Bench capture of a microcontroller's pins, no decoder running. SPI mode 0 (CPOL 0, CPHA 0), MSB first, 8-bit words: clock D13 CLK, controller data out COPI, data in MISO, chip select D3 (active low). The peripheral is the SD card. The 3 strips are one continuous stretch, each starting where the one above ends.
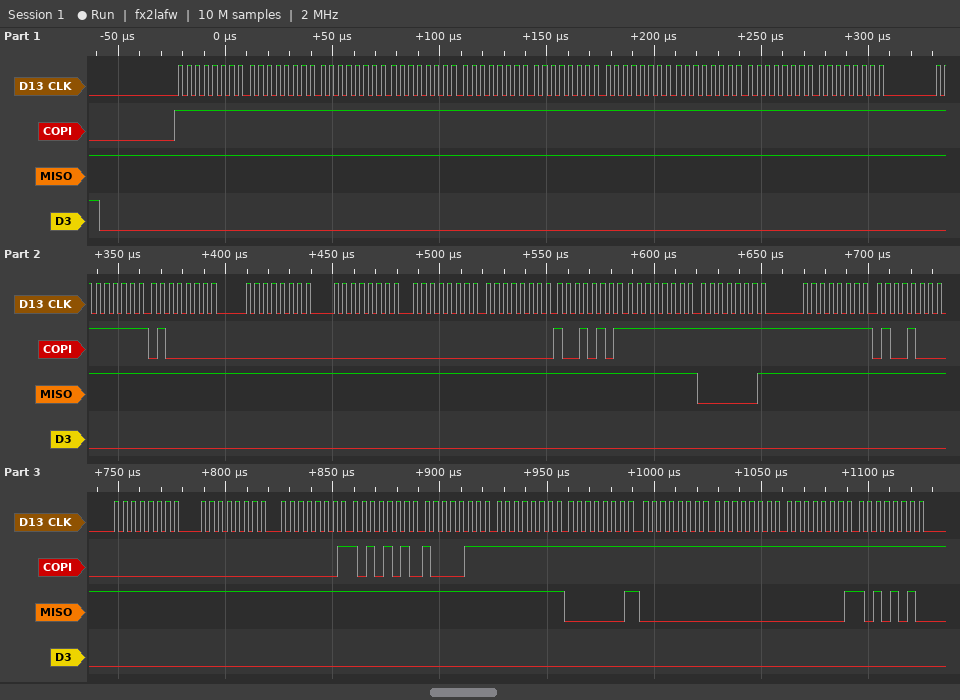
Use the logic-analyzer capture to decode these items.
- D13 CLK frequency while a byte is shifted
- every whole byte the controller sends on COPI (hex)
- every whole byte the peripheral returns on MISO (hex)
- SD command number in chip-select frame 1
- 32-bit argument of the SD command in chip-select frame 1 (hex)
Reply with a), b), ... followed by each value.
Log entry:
a) 250 kHz
b) 0xFF 0xFF 0xFF 0xFF 0xFF 0xFF 0xFF 0xFF 0xFF 0xFF 0xFF 0x40 0x00 0x00 0x00 0x00 0x95 0xFF 0xFF 0xFF 0x48 0x00 0x00 0x01 0xAA 0x87 0xFF 0xFF 0xFF 0xFF 0xFF 0xFF
c) 0xFF 0xFF 0xFF 0xFF 0xFF 0xFF 0xFF 0xFF 0xFF 0xFF 0xFF 0xFF 0xFF 0xFF 0xFF 0xFF 0xFF 0xFF 0x01 0xFF 0xFF 0xFF 0xFF 0xFF 0xFF 0xFF 0xFF 0x01 0x00 0x00 0x01 0xAA
d) CMD0
e) 0x00000000
